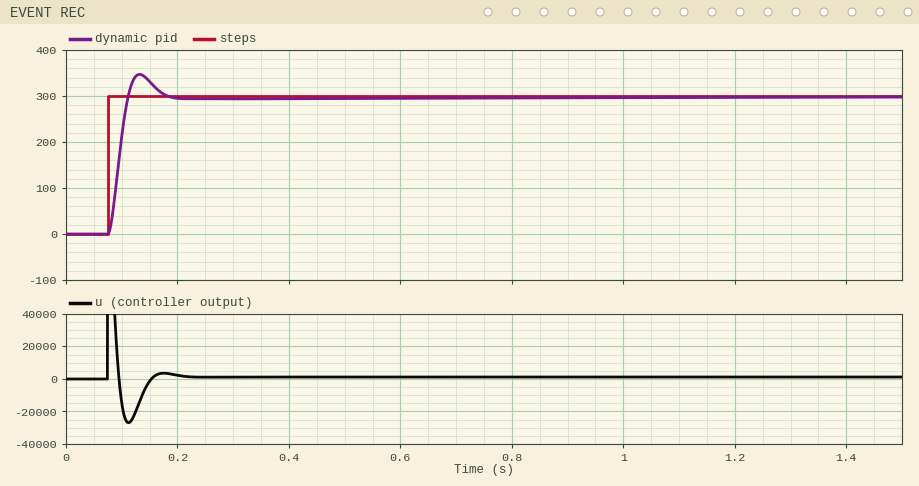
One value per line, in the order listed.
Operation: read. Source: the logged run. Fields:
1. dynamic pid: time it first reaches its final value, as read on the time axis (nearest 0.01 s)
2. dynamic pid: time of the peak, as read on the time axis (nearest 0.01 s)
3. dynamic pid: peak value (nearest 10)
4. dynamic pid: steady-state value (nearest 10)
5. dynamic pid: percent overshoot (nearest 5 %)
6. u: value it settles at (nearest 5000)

0.11 s
0.13 s
350
300
15 %
0
